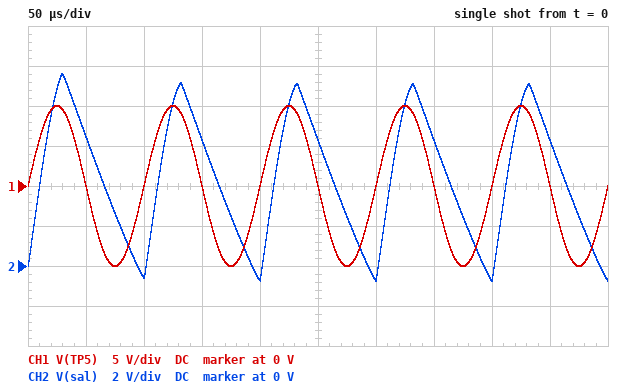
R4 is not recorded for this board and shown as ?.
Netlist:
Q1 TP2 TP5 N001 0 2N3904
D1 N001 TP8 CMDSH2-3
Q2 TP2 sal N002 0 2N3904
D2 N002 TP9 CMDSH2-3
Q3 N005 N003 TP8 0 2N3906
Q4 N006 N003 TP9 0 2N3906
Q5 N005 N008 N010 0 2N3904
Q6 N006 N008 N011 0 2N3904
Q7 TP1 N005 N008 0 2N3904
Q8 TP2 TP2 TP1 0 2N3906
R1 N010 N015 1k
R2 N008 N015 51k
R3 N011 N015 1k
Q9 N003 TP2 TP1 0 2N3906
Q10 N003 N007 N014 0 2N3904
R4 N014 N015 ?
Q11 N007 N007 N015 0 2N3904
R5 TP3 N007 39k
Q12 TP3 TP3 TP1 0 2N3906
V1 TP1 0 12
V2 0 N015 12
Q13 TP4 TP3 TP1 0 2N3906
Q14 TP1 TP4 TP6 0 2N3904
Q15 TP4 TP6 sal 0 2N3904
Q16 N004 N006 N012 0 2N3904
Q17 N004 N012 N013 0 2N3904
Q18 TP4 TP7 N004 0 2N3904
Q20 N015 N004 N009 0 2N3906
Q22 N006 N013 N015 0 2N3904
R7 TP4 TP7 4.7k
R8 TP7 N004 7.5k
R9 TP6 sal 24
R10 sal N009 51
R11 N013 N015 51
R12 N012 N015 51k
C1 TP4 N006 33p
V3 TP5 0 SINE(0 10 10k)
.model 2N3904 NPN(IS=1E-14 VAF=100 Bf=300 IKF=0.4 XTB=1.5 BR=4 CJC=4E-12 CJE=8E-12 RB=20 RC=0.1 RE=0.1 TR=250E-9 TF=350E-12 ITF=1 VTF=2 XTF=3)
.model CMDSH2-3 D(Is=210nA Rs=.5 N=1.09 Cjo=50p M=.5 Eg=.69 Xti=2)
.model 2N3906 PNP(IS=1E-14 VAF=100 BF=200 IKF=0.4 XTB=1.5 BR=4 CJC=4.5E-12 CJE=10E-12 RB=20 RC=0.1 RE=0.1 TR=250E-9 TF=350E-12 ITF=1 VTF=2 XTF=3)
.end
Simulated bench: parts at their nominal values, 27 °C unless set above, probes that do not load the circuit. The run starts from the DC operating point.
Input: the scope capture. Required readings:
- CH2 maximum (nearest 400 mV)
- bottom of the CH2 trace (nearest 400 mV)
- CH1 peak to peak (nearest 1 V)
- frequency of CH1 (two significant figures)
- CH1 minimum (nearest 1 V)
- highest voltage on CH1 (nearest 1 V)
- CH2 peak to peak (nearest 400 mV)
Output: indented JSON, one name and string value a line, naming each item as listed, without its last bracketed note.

{
  "CH2 maximum": "9.6 V",
  "bottom of the CH2 trace": "-800 mV",
  "CH1 peak to peak": "20 V",
  "frequency of CH1": "10 kHz",
  "CH1 minimum": "-10 V",
  "highest voltage on CH1": "10 V",
  "CH2 peak to peak": "10.4 V"
}
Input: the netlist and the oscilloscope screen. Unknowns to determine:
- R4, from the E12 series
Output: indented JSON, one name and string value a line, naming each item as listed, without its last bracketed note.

{
  "R4, from the E12 series": "15 kΩ"
}
